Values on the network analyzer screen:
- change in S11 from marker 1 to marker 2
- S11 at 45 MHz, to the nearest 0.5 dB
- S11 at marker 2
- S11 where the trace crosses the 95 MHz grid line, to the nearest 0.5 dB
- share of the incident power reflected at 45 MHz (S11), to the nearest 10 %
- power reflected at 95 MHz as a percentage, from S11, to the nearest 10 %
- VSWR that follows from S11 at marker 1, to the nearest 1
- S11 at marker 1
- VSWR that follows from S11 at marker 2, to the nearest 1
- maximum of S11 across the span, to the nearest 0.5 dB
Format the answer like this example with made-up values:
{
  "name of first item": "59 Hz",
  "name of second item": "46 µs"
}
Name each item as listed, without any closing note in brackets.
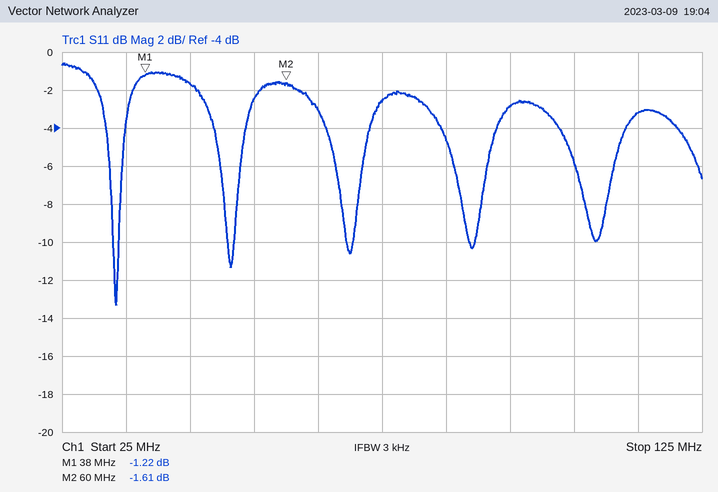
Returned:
{
  "change in S11 from marker 1 to marker 2": "-0.39 dB",
  "S11 at 45 MHz, to the nearest 0.5 dB": "-1.5 dB",
  "S11 at marker 2": "-1.61 dB",
  "S11 where the trace crosses the 95 MHz grid line, to the nearest 0.5 dB": "-3.0 dB",
  "share of the incident power reflected at 45 MHz (S11), to the nearest 10 %": "70 %",
  "power reflected at 95 MHz as a percentage, from S11, to the nearest 10 %": "50 %",
  "VSWR that follows from S11 at marker 1, to the nearest 1": "14",
  "S11 at marker 1": "-1.22 dB",
  "VSWR that follows from S11 at marker 2, to the nearest 1": "11",
  "maximum of S11 across the span, to the nearest 0.5 dB": "-0.5 dB"
}
